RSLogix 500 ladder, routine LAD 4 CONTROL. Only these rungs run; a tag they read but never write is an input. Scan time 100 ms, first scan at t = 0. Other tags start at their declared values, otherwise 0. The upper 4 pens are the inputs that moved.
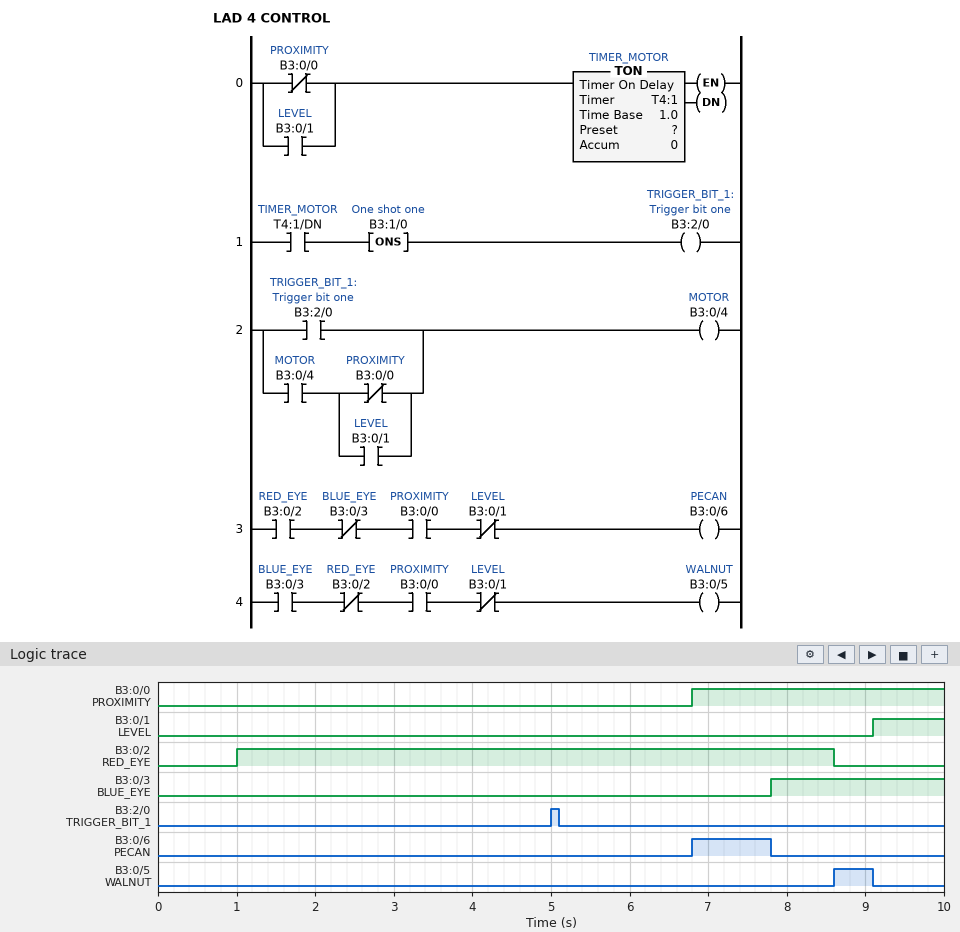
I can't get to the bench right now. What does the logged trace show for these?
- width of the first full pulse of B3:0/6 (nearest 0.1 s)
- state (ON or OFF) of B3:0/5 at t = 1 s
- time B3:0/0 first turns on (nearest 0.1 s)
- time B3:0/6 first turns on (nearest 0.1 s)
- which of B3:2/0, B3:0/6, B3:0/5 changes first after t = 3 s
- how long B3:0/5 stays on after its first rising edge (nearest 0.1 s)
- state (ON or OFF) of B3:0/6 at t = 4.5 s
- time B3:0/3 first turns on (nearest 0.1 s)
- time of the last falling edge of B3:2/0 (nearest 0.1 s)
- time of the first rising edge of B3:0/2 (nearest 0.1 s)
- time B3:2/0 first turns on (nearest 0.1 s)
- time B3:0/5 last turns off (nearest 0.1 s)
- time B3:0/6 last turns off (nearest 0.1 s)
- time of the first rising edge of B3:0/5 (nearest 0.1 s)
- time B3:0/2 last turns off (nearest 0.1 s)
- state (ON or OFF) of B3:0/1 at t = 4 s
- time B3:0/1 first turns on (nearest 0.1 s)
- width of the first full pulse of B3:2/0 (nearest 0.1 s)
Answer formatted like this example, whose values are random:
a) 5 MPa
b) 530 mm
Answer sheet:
a) 1.0 s
b) OFF
c) 6.8 s
d) 6.8 s
e) B3:2/0
f) 0.5 s
g) OFF
h) 7.8 s
i) 5.1 s
j) 1.0 s
k) 5.0 s
l) 9.1 s
m) 7.8 s
n) 8.6 s
o) 8.6 s
p) OFF
q) 9.1 s
r) 0.1 s
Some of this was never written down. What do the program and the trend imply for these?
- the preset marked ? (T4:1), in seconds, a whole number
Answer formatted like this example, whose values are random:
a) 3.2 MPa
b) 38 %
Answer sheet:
a) 5 s
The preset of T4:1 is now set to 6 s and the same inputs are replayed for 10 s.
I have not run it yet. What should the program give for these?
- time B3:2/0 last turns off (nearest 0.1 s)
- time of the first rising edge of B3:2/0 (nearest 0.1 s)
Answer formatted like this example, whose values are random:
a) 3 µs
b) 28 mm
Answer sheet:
a) 6.1 s
b) 6.0 s
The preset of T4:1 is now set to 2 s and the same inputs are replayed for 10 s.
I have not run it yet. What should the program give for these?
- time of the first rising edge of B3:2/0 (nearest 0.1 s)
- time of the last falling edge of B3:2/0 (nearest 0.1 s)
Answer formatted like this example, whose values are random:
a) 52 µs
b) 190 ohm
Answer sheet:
a) 2.0 s
b) 2.1 s
